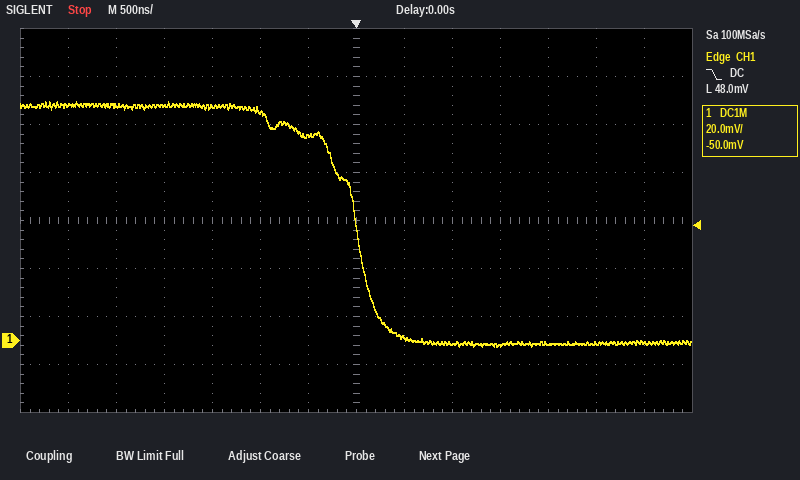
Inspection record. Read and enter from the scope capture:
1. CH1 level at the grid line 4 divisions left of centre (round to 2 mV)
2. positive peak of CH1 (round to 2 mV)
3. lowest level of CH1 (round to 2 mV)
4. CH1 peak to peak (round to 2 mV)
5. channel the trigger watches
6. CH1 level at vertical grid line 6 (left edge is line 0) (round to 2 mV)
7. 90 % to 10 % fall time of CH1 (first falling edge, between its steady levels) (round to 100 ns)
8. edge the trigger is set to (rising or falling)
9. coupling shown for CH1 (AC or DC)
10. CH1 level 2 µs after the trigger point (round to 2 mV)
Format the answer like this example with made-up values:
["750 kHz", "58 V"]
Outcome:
["98 mV", "100 mV", "-2 mV", "102 mV", "CH1", "86 mV", "900 ns", "falling", "DC", "-2 mV"]
